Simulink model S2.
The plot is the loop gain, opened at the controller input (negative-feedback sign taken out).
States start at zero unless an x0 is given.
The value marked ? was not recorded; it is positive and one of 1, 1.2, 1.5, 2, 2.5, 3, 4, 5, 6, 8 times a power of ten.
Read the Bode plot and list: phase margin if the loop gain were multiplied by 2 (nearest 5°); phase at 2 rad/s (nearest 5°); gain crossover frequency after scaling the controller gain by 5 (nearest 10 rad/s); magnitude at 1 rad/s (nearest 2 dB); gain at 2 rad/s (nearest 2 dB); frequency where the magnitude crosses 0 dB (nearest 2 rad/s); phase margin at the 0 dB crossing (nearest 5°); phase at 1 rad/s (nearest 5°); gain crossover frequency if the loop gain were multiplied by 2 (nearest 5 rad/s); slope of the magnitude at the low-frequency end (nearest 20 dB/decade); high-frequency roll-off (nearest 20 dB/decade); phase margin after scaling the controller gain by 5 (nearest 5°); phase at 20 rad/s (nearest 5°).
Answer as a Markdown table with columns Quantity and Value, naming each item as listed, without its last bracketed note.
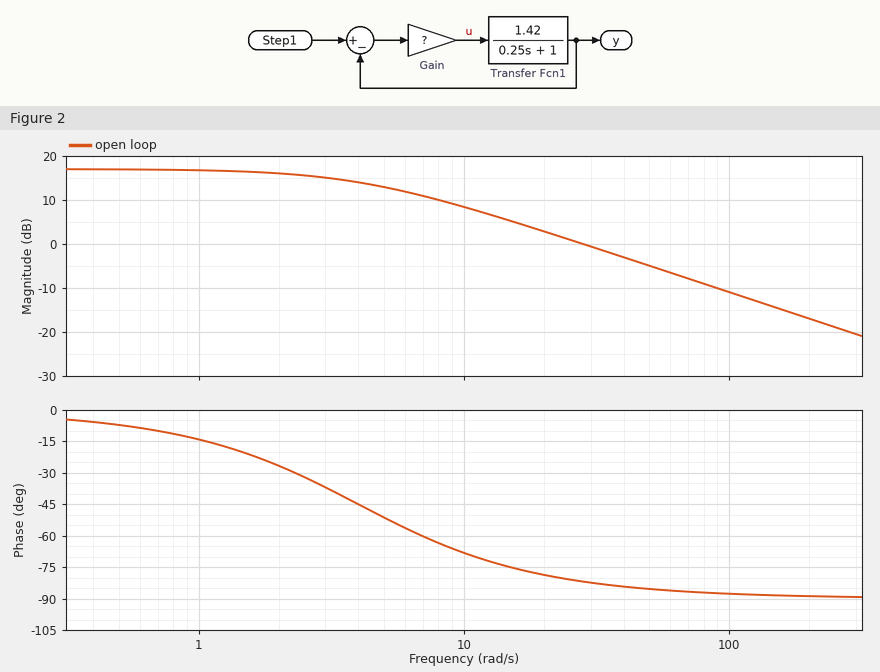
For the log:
| Quantity | Value |
|---|---|
| phase margin if the loop gain were multiplied by 2 | 95° |
| phase at 2 rad/s | -25° |
| gain crossover frequency after scaling the controller gain by 5 | 140 rad/s |
| magnitude at 1 rad/s | 16 dB |
| gain at 2 rad/s | 16 dB |
| frequency where the magnitude crosses 0 dB | 28 rad/s |
| phase margin at the 0 dB crossing | 100° |
| phase at 1 rad/s | -15° |
| gain crossover frequency if the loop gain were multiplied by 2 | 55 rad/s |
| slope of the magnitude at the low-frequency end | 0 dB/decade |
| high-frequency roll-off | -20 dB/decade |
| phase margin after scaling the controller gain by 5 | 90° |
| phase at 20 rad/s | -80° |
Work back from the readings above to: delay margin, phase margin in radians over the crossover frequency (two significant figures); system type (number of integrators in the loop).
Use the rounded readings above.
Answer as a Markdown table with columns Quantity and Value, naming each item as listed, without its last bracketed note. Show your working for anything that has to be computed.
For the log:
| Quantity | Value |
|---|---|
| delay margin, phase margin in radians over the crossover frequency | 100 × π / 180 / 28 = 0.062 s |
| system type | 0 |
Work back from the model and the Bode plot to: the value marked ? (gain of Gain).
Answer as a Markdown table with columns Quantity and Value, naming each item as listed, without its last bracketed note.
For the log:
| Quantity | Value |
|---|---|
| the value marked ? | 5 |
